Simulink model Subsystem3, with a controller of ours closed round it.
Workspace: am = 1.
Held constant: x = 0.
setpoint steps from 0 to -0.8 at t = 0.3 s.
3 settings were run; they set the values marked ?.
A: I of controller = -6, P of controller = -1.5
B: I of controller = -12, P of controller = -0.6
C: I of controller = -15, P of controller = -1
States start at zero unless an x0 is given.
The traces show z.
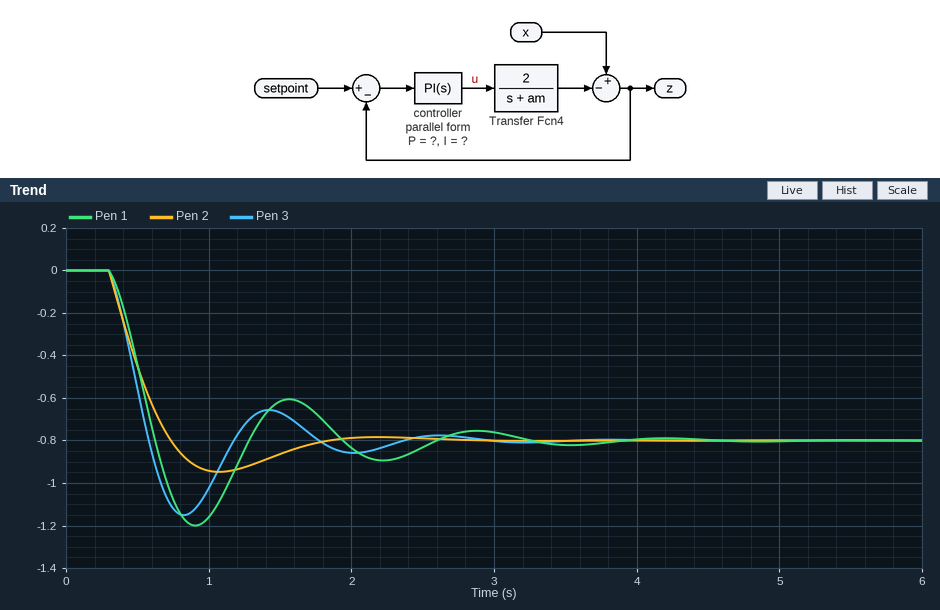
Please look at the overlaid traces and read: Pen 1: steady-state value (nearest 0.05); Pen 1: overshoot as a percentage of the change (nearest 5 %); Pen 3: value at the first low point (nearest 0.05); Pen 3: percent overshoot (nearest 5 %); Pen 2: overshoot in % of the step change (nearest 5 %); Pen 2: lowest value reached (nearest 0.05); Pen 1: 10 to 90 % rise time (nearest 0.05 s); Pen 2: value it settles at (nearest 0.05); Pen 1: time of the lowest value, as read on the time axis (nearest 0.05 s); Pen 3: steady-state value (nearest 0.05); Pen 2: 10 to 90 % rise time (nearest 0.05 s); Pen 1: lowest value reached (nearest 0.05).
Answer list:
-0.80
50 %
-1.15
45 %
20 %
-0.95
0.25 s
-0.80
0.90 s
-0.80
0.35 s
-1.20
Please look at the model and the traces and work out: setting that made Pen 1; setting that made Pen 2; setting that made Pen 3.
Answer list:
B
A
C
